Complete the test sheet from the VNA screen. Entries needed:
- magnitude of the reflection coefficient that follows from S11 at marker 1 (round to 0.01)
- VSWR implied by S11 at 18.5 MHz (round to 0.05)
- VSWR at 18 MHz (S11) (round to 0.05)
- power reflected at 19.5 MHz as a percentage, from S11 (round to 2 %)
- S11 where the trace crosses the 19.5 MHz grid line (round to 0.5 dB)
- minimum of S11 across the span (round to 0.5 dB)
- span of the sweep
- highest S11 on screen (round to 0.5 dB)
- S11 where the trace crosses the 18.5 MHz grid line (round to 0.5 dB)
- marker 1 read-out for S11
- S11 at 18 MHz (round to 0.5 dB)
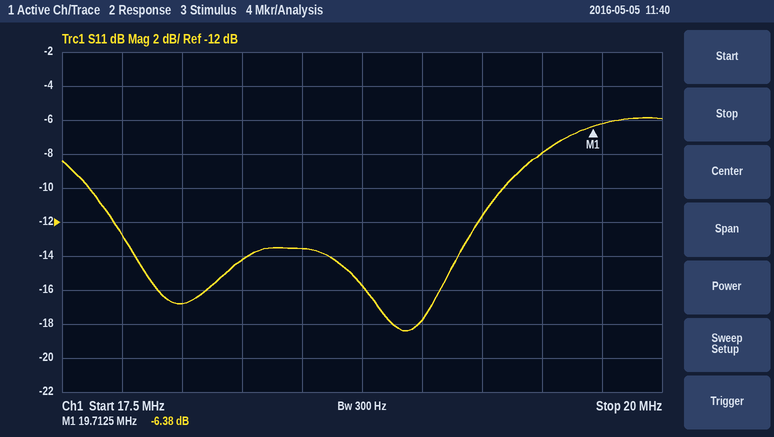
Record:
0.48
1.55
1.35
16 %
-8.0 dB
-18.5 dB
2.5 MHz
-6.0 dB
-13.5 dB
-6.38 dB
-17.0 dB
